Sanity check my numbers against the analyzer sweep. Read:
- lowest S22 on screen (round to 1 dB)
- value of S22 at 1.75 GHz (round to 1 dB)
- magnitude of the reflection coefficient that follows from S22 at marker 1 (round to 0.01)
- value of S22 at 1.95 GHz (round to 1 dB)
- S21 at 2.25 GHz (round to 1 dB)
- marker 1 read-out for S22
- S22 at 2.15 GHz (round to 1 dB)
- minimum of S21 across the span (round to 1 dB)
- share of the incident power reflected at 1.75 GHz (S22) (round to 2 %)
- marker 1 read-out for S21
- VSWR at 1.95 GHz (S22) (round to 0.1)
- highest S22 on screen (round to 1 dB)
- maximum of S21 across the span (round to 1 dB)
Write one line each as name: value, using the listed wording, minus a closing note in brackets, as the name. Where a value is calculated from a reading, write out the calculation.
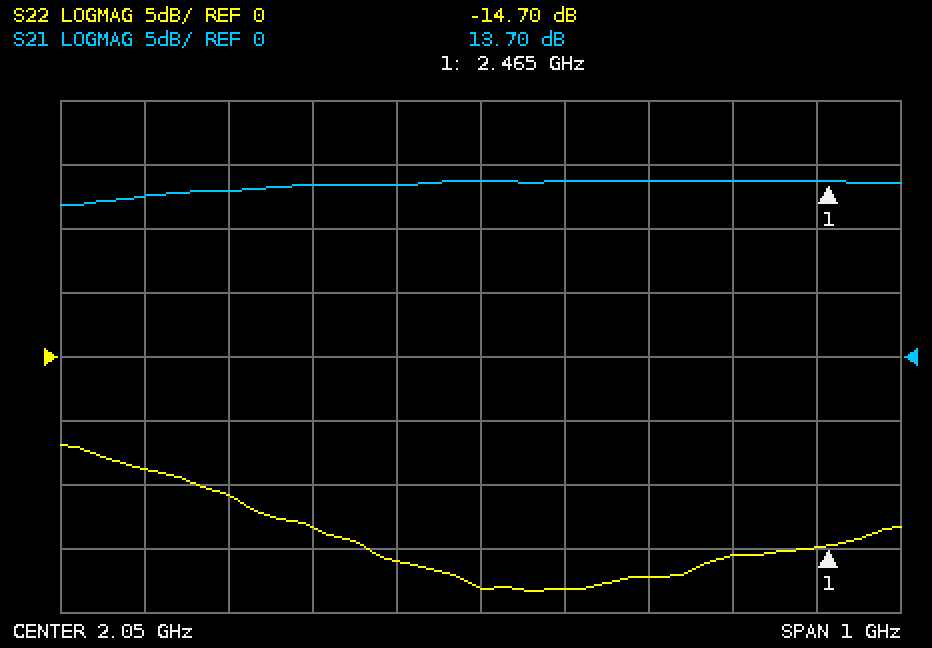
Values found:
lowest S22 on screen: -18 dB
value of S22 at 1.75 GHz: -11 dB
magnitude of the reflection coefficient that follows from S22 at marker 1: 10^(-14.7/20) ≈ 0.18
value of S22 at 1.95 GHz: -16 dB
S21 at 2.25 GHz: 14 dB
marker 1 read-out for S22: -14.70 dB
S22 at 2.15 GHz: -18 dB
minimum of S21 across the span: 12 dB
share of the incident power reflected at 1.75 GHz (S22): 10^(-11/10) ≈ 8 %
marker 1 read-out for S21: 13.70 dB
VSWR at 1.95 GHz (S22): |Γ| = 10^(-16/20) = 0.1585; VSWR = (1 + 0.1585)/(1 − 0.1585) ≈ 1.4
highest S22 on screen: -7 dB
maximum of S21 across the span: 14 dB
